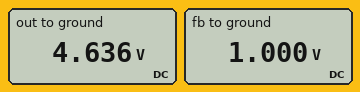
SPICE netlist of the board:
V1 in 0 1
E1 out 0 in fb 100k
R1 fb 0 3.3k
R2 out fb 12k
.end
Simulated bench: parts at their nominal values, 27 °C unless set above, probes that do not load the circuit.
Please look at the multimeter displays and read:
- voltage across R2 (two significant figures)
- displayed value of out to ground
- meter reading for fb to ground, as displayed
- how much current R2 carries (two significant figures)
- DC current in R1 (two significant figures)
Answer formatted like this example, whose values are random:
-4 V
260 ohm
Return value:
3.6 V
4.636 V
1.000 V
300 µA
300 µA
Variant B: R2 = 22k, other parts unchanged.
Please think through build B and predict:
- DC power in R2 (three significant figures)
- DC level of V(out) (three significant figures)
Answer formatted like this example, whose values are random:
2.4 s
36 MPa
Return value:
2.02 mW
7.67 V
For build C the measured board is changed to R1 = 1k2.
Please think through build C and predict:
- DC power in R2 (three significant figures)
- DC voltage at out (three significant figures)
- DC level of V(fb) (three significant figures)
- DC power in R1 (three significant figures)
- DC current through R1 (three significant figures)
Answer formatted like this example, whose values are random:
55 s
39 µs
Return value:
8.33 mW
11.0 V
1.00 V
833 µW
833 µA
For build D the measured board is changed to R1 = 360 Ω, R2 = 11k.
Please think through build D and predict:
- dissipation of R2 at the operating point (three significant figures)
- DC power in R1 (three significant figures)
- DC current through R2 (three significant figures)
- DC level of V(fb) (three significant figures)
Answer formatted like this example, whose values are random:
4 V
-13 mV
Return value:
84.8 mW
2.78 mW
2.78 mA
1.00 V
